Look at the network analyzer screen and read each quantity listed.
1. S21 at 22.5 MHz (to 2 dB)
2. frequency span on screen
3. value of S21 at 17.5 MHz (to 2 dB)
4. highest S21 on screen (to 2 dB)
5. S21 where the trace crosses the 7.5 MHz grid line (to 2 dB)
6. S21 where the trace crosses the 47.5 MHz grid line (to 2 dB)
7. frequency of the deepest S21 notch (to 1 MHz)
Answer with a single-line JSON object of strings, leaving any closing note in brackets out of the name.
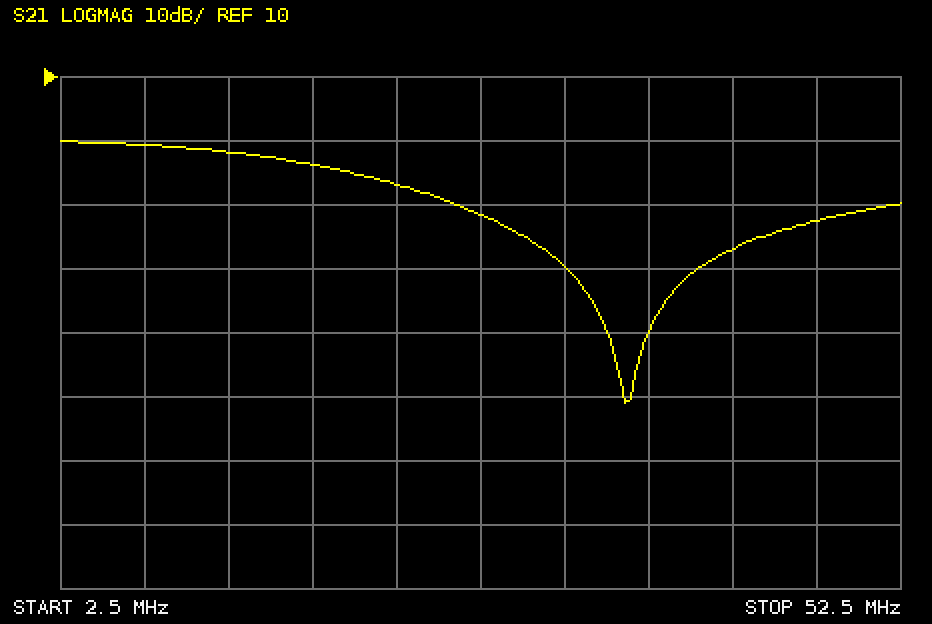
{"S21 at 22.5 MHz": "-6 dB", "frequency span on screen": "50 MHz", "value of S21 at 17.5 MHz": "-4 dB", "highest S21 on screen": "0 dB", "S21 where the trace crosses the 7.5 MHz grid line": "0 dB", "S21 where the trace crosses the 47.5 MHz grid line": "-12 dB", "frequency of the deepest S21 notch": "36 MHz"}
